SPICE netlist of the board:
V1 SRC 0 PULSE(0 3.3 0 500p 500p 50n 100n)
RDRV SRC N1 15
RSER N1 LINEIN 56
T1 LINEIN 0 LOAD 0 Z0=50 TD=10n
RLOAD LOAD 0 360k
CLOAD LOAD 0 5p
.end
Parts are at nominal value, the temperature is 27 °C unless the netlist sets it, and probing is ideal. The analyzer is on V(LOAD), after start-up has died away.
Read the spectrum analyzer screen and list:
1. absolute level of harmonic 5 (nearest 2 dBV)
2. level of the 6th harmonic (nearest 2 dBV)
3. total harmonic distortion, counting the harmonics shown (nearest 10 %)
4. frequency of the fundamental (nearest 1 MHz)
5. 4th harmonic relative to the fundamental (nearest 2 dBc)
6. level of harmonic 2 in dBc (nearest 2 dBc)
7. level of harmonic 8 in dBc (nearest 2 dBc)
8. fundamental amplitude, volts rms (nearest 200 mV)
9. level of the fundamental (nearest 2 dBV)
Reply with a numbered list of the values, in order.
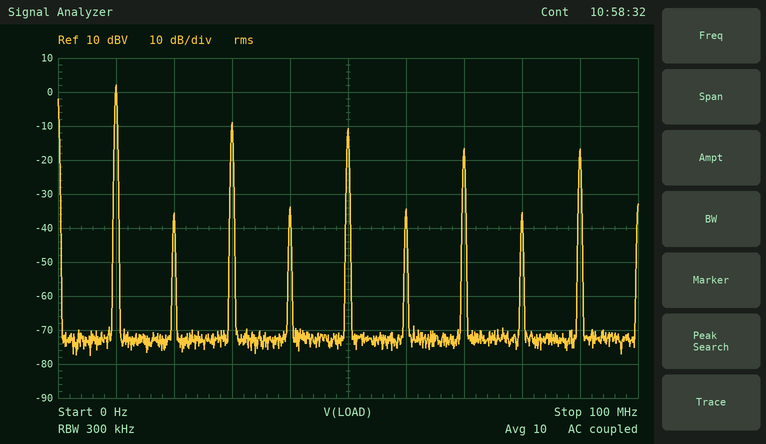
1. -10 dBV
2. -34 dBV
3. 40 %
4. 10 MHz
5. -36 dBc
6. -38 dBc
7. -38 dBc
8. 1.2 V
9. 2 dBV
